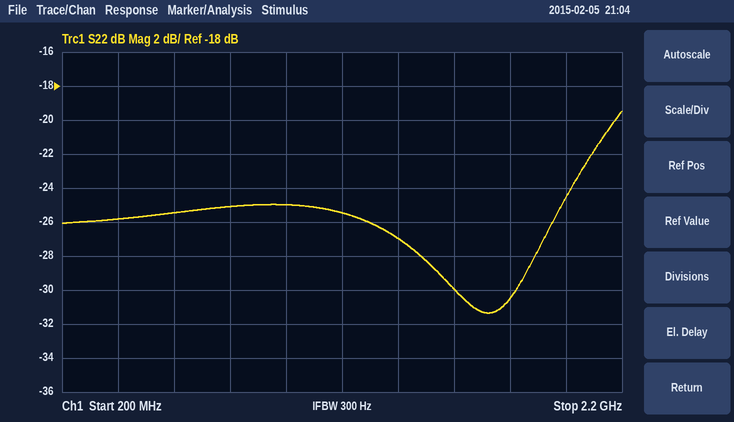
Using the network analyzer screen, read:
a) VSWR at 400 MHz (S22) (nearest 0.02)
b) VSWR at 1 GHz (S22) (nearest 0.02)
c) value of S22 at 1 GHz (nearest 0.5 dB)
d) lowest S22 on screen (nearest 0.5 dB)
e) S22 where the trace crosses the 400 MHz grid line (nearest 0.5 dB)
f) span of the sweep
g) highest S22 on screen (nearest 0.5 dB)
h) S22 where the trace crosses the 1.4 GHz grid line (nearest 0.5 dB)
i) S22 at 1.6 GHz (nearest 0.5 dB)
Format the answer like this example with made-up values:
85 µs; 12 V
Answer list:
1.10; 1.12; -25.0 dB; -31.5 dB; -26.0 dB; 2 GHz; -19.5 dB; -27.0 dB; -30.0 dB
